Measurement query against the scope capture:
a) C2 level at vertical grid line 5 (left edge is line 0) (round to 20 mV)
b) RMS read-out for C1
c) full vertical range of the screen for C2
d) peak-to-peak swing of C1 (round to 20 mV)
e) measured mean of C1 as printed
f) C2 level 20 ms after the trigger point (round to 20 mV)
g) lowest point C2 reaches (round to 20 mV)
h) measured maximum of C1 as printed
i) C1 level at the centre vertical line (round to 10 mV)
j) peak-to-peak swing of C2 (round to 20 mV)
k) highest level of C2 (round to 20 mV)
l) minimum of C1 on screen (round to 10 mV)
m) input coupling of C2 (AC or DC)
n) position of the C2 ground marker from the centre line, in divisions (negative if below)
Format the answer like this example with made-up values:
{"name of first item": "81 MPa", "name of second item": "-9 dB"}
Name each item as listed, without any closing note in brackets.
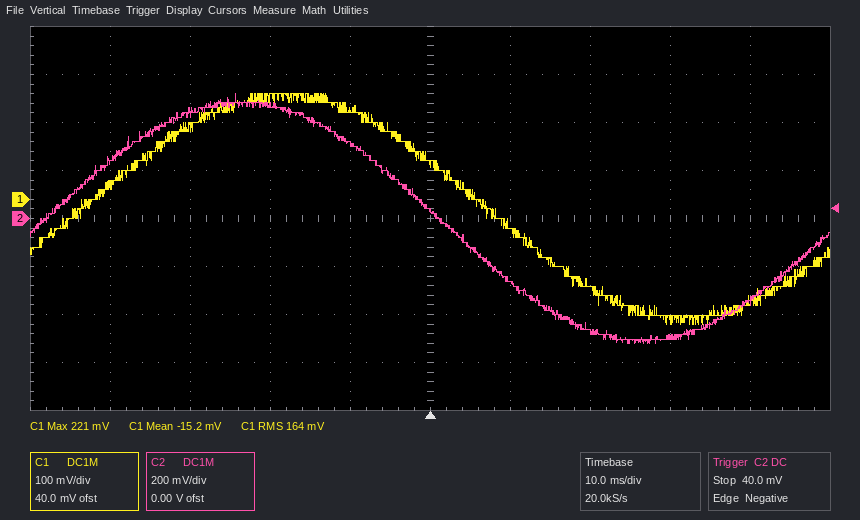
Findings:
{"C2 level at vertical grid line 5 (left edge is line 0)": "40 mV", "RMS read-out for C1": "164 mV", "full vertical range of the screen for C2": "1.6 V", "peak-to-peak swing of C1": "480 mV", "measured mean of C1 as printed": "-15.2 mV", "C2 level 20 ms after the trigger point": "-480 mV", "lowest point C2 reaches": "-520 mV", "measured maximum of C1 as printed": "221 mV", "C1 level at the centre vertical line": "70 mV", "peak-to-peak swing of C2": "1.04 V", "highest level of C2": "520 mV", "minimum of C1 on screen": "-260 mV", "input coupling of C2": "DC", "position of the C2 ground marker from the centre line, in divisions": "0.0 div"}
